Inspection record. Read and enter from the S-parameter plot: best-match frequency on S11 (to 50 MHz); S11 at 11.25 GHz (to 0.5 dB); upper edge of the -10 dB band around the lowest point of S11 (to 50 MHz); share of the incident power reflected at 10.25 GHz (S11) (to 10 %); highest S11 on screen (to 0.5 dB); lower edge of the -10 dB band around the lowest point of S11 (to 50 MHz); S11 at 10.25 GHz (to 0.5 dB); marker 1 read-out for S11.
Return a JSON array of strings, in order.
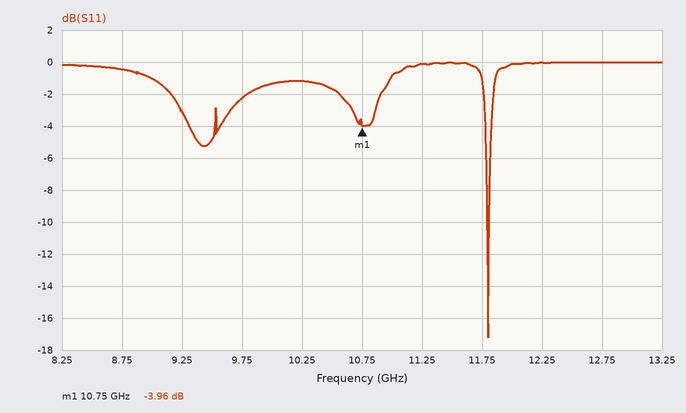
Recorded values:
["11.80 GHz", "0.0 dB", "11.80 GHz", "80 %", "0.0 dB", "11.80 GHz", "-1.0 dB", "-3.96 dB"]
